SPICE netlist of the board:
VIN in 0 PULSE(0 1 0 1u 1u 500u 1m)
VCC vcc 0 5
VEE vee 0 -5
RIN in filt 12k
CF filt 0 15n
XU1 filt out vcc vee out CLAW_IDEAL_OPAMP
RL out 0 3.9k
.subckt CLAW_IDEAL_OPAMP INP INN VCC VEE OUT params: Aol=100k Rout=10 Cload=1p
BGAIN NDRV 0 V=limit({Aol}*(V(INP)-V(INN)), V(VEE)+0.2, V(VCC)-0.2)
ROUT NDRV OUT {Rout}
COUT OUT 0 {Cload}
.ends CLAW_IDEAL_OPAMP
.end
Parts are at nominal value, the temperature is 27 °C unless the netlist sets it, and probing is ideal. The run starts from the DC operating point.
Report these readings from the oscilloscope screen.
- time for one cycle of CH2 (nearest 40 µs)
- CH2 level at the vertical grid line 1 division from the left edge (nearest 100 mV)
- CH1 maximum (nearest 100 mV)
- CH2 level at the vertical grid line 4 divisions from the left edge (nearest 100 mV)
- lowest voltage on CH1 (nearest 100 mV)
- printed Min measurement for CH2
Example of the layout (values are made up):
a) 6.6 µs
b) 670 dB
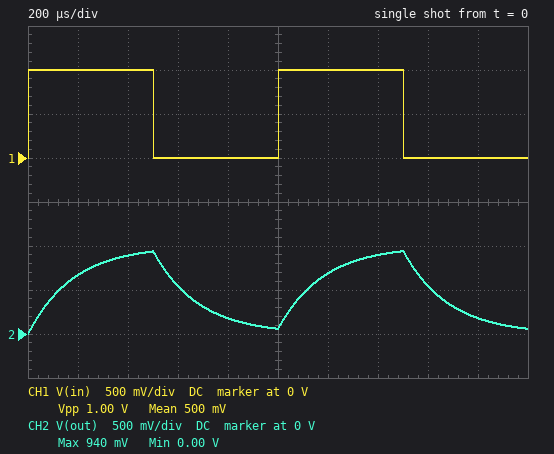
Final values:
a) 1.00 ms
b) 700 mV
c) 1.0 V
d) 200 mV
e) 0 V
f) 0.00 V
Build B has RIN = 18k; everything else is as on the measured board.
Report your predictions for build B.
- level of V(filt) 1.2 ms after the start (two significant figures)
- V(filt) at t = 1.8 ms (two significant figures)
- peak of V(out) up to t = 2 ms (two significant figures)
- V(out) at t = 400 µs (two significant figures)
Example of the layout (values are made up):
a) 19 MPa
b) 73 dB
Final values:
a) 590 mV
b) 290 mV
c) 860 mV
d) 770 mV
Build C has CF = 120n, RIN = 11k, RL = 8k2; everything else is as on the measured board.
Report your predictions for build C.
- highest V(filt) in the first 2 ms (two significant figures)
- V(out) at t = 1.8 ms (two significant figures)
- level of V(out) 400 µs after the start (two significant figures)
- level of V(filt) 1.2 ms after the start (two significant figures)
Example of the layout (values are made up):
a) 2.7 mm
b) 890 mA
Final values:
a) 460 mV
b) 370 mV
c) 260 mV
d) 330 mV
